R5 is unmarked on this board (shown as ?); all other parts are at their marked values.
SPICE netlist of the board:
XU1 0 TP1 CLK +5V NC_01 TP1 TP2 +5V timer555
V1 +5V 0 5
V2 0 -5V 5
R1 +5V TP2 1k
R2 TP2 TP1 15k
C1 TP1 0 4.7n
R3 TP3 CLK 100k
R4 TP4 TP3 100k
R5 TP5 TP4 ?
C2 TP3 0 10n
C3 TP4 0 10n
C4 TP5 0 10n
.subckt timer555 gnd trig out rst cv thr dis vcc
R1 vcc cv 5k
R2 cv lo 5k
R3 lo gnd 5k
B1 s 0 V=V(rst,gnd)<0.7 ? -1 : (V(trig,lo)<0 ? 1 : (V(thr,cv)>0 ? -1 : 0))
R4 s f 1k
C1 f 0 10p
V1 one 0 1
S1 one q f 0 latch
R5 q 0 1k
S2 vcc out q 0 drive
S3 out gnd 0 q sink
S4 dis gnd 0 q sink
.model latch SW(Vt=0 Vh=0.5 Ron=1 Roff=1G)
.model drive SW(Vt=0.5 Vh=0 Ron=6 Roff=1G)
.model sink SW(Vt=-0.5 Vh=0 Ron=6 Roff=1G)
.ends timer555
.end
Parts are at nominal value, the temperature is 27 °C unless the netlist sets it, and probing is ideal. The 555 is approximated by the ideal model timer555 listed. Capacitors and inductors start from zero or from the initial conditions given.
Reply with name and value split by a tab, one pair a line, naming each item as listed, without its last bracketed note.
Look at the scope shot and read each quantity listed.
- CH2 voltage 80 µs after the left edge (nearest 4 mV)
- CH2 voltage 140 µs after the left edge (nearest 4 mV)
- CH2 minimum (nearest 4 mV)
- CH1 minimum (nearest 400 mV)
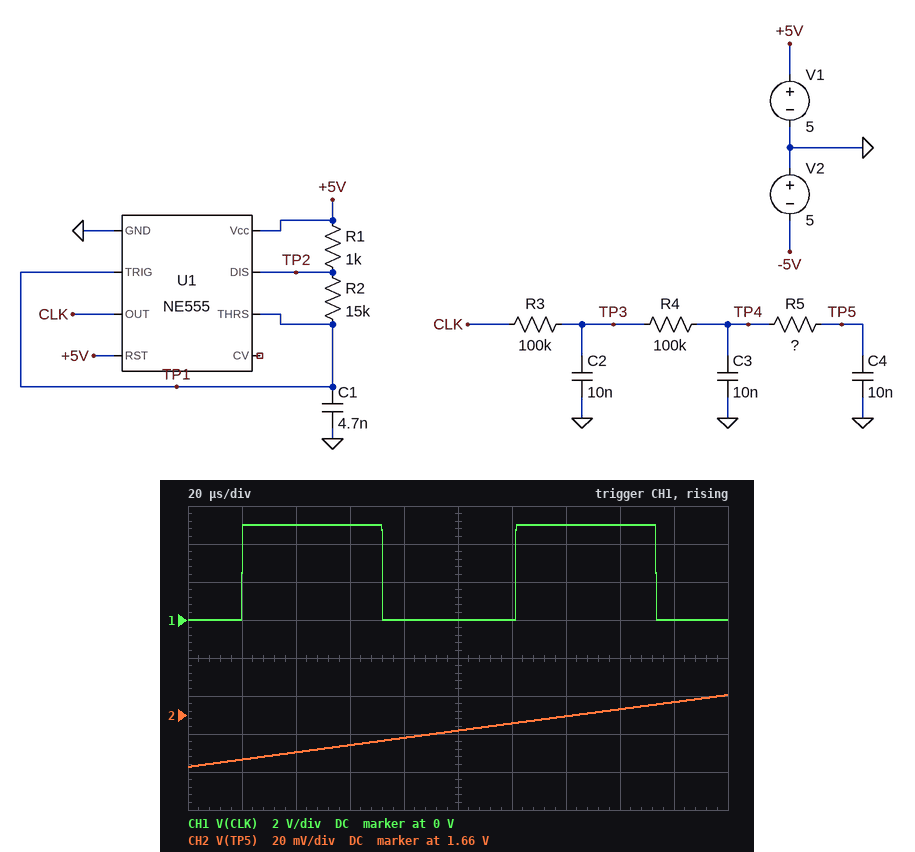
CH2 voltage 80 µs after the left edge	1.648 V
CH2 voltage 140 µs after the left edge	1.660 V
CH2 minimum	1.632 V
CH1 minimum	0 V
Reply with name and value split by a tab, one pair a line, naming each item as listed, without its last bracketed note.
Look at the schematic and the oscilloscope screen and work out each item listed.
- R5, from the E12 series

R5, from the E12 series	56 kΩ
